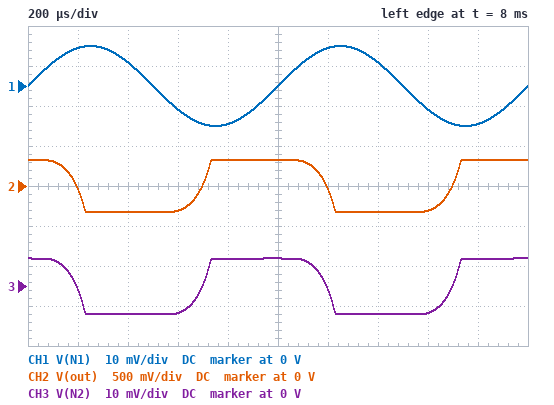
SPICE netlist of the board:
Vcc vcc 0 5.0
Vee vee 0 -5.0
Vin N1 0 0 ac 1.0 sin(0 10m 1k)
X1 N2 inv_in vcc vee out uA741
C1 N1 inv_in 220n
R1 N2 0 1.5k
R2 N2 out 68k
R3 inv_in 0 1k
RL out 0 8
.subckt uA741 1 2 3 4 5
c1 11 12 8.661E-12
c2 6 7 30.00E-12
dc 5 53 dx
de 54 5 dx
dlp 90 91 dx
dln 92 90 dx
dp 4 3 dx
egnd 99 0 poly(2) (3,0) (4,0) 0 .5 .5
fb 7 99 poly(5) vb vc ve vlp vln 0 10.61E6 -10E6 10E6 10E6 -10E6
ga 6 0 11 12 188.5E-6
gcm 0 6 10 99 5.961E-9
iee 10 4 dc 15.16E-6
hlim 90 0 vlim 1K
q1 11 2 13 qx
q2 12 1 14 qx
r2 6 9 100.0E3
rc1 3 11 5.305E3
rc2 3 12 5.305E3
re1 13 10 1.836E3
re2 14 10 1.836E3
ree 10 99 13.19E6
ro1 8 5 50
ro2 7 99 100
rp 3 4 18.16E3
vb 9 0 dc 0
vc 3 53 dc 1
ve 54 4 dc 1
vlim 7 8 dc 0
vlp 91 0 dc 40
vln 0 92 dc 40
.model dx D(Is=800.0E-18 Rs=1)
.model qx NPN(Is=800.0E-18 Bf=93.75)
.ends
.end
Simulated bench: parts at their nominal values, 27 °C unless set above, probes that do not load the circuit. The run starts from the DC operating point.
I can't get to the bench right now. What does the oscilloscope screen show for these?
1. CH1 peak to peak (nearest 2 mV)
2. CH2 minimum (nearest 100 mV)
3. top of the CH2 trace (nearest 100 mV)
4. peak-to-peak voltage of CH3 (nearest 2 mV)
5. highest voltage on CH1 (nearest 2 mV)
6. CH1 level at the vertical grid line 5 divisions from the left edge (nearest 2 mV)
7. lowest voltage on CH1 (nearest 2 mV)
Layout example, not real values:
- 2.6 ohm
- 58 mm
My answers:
- 20 mV
- -300 mV
- 300 mV
- 14 mV
- 10 mV
- 0 V
- -10 mV
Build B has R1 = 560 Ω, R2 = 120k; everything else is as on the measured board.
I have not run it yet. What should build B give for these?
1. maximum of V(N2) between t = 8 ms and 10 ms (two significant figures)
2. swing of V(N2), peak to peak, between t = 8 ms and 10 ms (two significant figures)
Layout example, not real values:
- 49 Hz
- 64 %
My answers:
- 1.5 mV
- 3.0 mV
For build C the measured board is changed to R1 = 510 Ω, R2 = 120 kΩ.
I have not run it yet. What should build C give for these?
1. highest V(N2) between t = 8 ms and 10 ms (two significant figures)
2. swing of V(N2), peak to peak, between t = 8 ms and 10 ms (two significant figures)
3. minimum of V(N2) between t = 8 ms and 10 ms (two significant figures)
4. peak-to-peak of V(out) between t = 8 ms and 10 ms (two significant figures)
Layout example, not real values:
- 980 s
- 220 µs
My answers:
- 1.3 mV
- 2.7 mV
- -1.4 mV
- 650 mV
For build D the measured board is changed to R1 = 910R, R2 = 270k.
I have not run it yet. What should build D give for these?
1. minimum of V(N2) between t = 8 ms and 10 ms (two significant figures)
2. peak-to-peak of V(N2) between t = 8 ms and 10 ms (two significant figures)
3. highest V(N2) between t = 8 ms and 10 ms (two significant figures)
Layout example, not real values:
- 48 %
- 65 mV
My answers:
- -1.2 mV
- 2.2 mV
- 1.0 mV
